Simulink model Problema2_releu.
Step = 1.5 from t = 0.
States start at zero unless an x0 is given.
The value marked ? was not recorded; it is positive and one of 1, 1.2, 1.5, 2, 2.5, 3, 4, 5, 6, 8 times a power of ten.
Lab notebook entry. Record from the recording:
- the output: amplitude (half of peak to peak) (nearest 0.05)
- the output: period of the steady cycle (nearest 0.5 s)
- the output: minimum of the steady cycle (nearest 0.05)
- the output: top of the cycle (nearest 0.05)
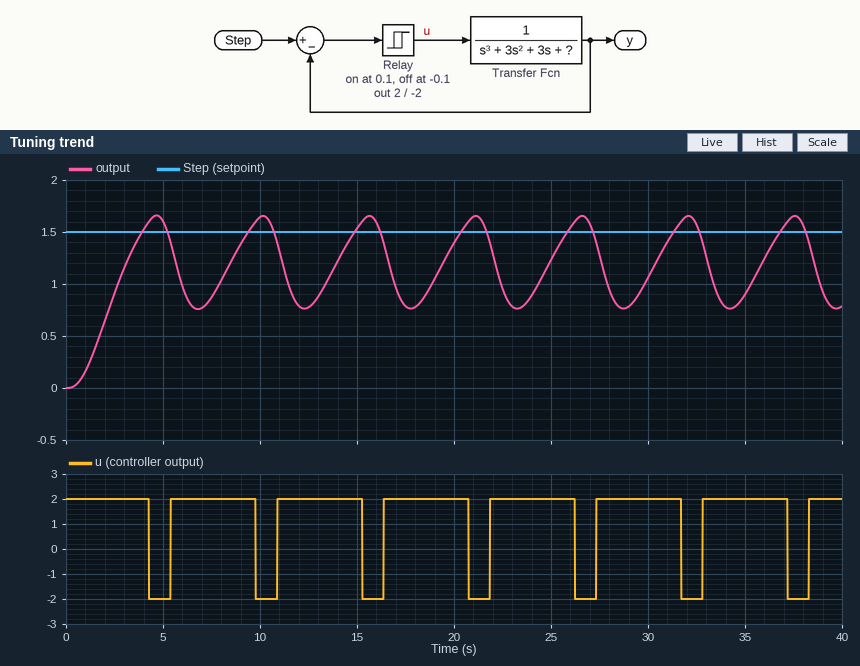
0.45
5.5 s
0.75
1.65
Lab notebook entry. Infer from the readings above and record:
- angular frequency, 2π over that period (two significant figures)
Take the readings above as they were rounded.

1.1 rad/s
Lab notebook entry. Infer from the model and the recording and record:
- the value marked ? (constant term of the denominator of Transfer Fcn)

1
